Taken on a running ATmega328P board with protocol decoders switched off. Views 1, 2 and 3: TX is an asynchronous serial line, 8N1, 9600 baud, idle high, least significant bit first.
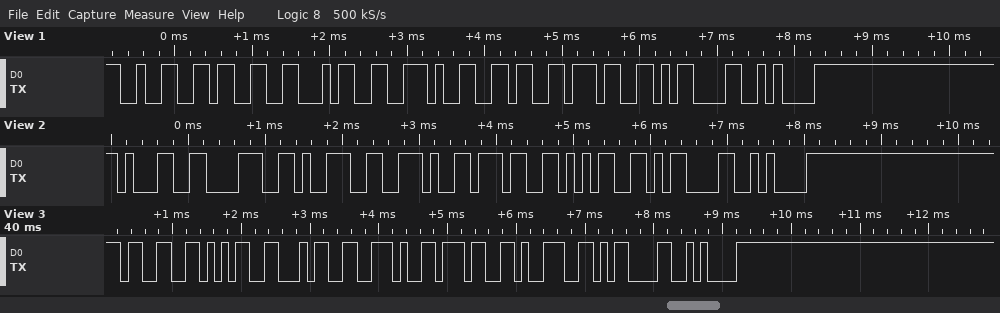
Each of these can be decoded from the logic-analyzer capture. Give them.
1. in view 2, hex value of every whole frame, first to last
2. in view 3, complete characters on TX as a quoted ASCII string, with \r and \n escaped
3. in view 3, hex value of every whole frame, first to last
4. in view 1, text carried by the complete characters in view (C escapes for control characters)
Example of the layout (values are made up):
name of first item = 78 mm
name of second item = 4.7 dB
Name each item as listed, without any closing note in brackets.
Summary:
in view 2, hex value of every whole frame, first to last = 31 38 39 2E 37 35 0D 0A
in view 3, complete characters on TX as a quoted ASCII string, with \r and \n escaped = "354.79\r\n"
in view 3, hex value of every whole frame, first to last = 0x33 0x35 0x34 0x2E 0x37 0x39 0x0D 0x0A
in view 1, text carried by the complete characters in view = "234.67\r\n"
